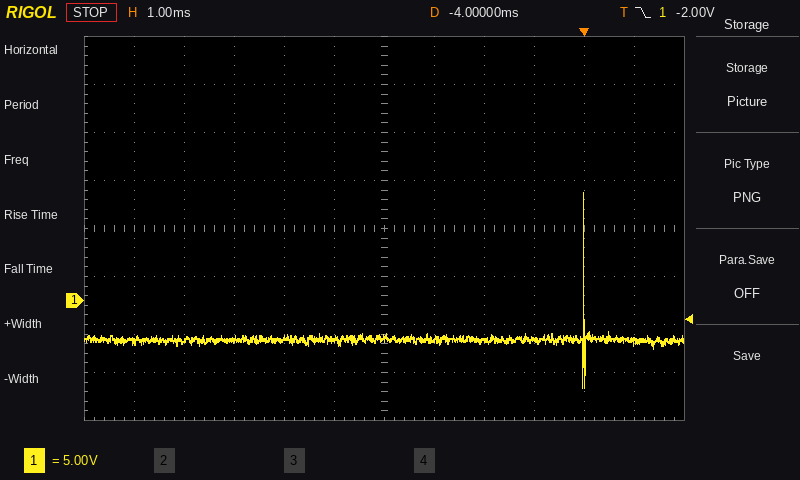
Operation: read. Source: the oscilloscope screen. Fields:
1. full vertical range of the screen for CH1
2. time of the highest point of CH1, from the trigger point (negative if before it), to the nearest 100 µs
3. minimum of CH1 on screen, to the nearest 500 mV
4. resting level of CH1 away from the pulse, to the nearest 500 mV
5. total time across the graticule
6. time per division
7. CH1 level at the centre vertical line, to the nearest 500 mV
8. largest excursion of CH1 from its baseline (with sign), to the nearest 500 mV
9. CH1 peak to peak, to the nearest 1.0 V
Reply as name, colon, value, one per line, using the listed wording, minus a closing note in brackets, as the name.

full vertical range of the screen for CH1: 40 V
time of the highest point of CH1, from the trigger point (negative if before it), to the nearest 100 µs: 0.0 ms
minimum of CH1 on screen, to the nearest 500 mV: -9.0 V
resting level of CH1 away from the pulse, to the nearest 500 mV: -4.0 V
total time across the graticule: 12 ms
time per division: 1 ms
CH1 level at the centre vertical line, to the nearest 500 mV: -4.0 V
largest excursion of CH1 from its baseline (with sign), to the nearest 500 mV: +15.5 V
CH1 peak to peak, to the nearest 1.0 V: 20.0 V
